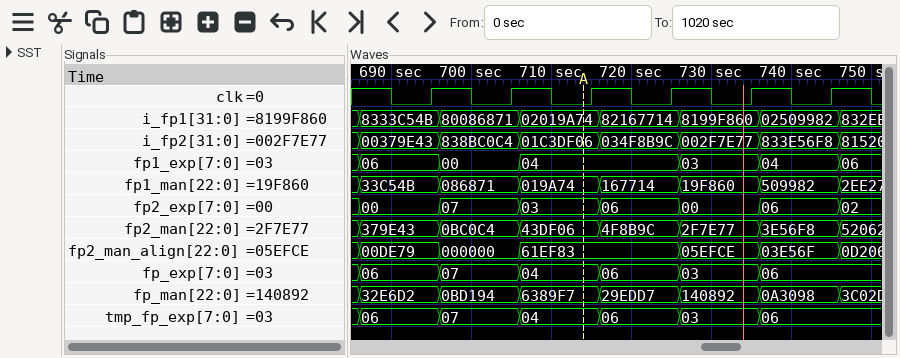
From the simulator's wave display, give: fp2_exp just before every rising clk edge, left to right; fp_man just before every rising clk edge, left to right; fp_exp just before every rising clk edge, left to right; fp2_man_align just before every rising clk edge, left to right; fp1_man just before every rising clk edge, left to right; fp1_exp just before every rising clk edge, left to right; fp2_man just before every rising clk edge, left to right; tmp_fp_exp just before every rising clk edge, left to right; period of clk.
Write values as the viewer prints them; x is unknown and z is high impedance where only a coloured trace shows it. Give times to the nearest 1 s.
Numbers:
00, 07, 03, 06, 00, 06
32E6D2, 0BD194, 6389F7, 29EDD7, 140892, 0A3098
06, 07, 04, 06, 03, 06
00DE79, 000000, 61EF83, 61EF83, 05EFCE, 03E56F
33C54B, 086871, 019A74, 167714, 19F860, 509982
06, 00, 04, 04, 03, 04
379E43, 0BC0C4, 43DF06, 4F8B9C, 2F7E77, 3E56F8
06, 07, 04, 06, 03, 06
10 s
